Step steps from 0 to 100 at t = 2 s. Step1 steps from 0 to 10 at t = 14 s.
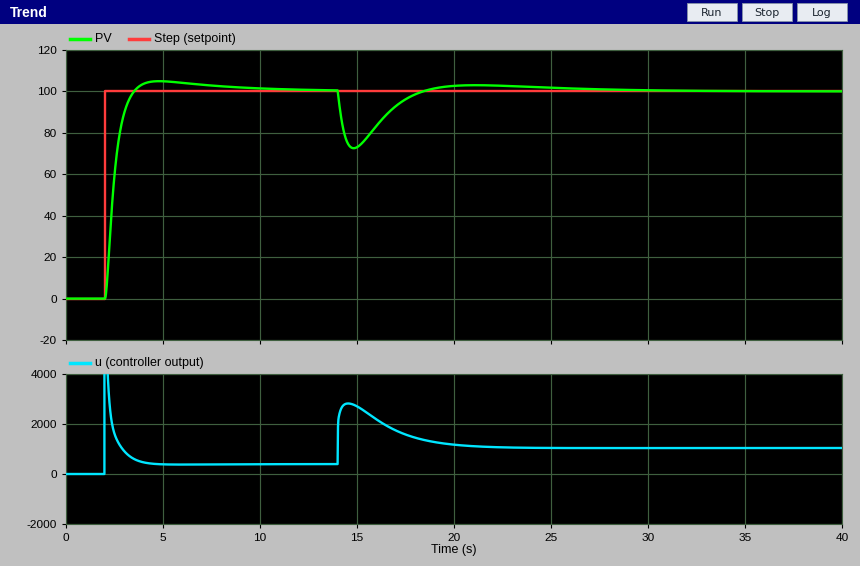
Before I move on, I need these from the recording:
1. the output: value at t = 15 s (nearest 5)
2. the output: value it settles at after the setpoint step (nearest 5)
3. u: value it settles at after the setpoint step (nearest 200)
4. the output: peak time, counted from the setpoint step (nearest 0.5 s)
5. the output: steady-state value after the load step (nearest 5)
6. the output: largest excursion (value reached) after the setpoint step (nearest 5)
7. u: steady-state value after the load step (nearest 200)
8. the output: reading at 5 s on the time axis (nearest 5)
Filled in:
75
100
400
3.0 s
100
105
1000
105
